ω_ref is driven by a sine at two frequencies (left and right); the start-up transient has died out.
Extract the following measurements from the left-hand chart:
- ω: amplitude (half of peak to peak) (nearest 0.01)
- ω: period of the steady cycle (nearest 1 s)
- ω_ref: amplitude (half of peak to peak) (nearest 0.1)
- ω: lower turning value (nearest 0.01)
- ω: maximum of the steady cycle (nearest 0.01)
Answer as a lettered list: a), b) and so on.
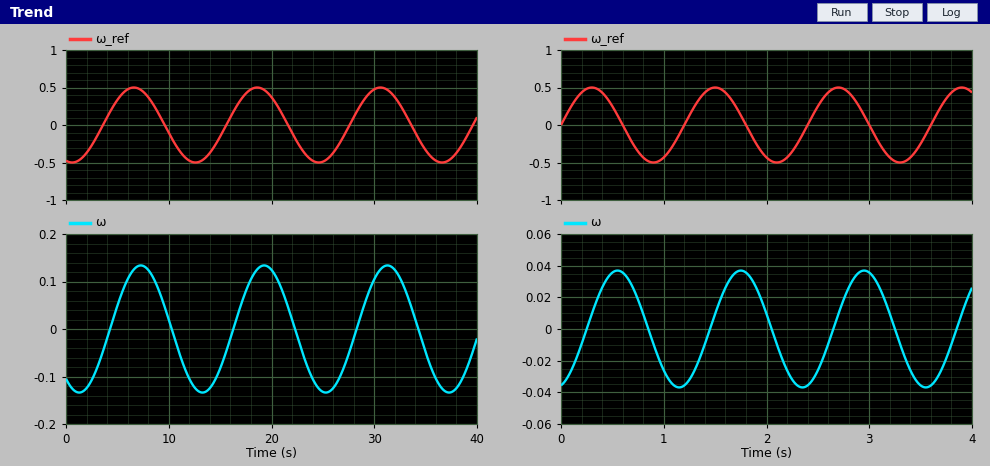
a) 0.13
b) 12 s
c) 0.5
d) -0.13
e) 0.13
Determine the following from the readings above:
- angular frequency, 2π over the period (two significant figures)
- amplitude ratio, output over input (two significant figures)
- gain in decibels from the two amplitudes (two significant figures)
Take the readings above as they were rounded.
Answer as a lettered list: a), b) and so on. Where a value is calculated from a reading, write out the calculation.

a) 2π / 12 = 0.52 rad/s
b) 0.13 / 0.5 = 0.26
c) 20 log10(0.13 / 0.5) = -12 dB
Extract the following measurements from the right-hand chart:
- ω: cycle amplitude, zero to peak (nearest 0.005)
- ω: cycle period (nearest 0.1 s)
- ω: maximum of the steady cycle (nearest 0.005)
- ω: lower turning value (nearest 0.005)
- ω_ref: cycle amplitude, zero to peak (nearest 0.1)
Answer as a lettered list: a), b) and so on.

a) 0.035
b) 1.2 s
c) 0.035
d) -0.035
e) 0.5
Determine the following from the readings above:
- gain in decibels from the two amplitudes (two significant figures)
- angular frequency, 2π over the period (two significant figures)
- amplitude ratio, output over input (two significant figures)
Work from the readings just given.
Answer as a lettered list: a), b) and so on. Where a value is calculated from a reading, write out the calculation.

a) 20 log10(0.035 / 0.5) = -23 dB
b) 2π / 1.2 = 5.2 rad/s
c) 0.035 / 0.5 = 0.070
